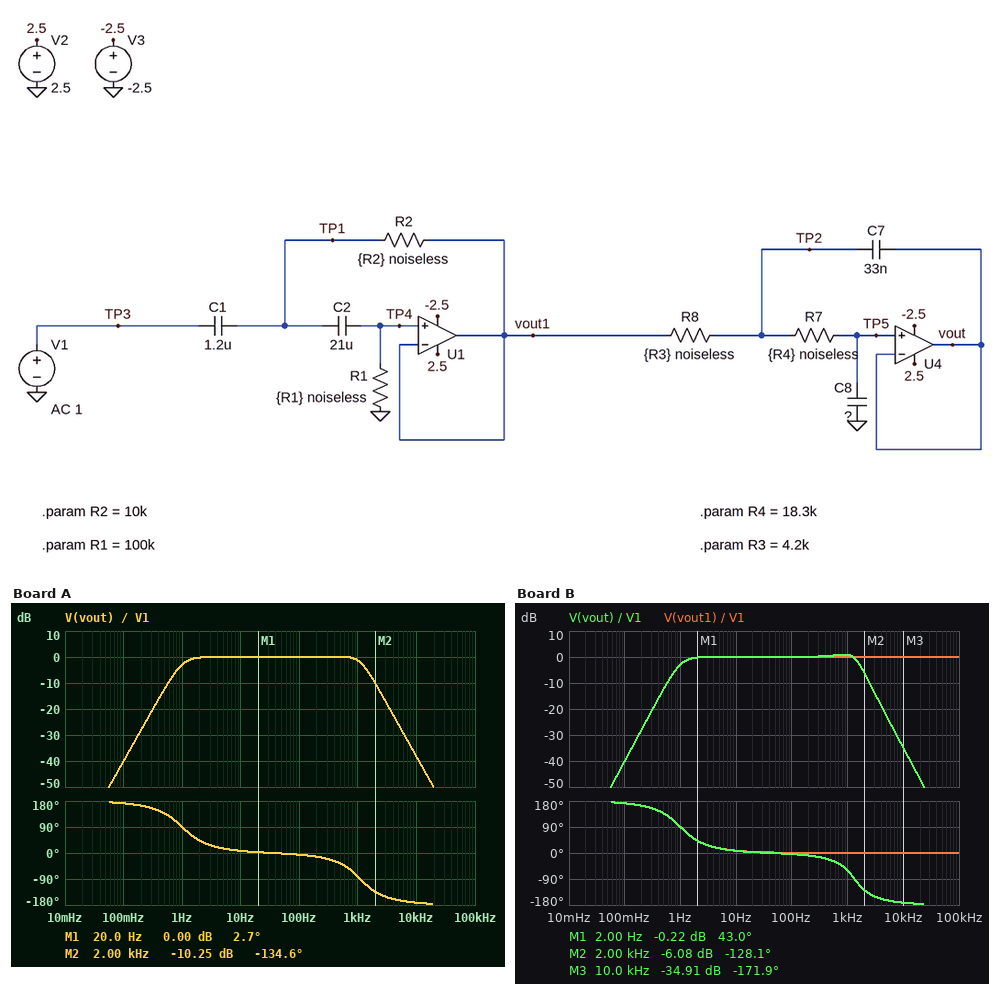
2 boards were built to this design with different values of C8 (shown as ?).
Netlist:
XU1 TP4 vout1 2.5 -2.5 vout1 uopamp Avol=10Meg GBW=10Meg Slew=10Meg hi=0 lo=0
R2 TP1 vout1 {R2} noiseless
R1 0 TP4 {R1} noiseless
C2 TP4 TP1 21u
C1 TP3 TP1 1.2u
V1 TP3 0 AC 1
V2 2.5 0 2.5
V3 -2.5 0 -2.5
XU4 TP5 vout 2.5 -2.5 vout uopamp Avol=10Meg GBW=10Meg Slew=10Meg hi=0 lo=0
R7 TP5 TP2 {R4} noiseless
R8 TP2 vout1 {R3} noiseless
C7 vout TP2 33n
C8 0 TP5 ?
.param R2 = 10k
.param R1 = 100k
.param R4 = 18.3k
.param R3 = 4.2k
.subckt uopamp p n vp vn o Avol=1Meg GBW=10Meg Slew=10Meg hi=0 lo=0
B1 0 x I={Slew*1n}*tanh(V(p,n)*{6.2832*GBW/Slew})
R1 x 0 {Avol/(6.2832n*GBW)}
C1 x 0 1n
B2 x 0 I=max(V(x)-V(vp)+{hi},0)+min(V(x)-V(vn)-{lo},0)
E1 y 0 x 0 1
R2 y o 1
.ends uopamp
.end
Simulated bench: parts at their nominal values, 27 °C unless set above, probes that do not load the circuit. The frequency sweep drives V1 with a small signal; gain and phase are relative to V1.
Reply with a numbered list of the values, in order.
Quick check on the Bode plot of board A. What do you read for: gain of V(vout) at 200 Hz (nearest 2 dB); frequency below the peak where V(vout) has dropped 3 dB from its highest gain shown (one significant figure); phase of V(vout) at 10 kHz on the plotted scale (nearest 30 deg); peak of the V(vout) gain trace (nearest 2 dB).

1. 0 dB
2. 1 Hz
3. -180 deg
4. 0 dB
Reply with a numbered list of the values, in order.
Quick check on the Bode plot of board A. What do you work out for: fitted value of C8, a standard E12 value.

1. 8.2 nF
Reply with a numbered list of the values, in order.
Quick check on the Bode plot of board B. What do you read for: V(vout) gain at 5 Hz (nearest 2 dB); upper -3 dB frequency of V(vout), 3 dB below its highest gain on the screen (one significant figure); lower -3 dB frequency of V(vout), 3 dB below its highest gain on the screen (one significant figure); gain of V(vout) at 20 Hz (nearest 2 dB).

1. 0 dB
2. 2 kHz
3. 1 Hz
4. 0 dB
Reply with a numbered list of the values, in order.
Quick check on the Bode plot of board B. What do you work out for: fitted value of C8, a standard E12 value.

1. 5.6 nF
